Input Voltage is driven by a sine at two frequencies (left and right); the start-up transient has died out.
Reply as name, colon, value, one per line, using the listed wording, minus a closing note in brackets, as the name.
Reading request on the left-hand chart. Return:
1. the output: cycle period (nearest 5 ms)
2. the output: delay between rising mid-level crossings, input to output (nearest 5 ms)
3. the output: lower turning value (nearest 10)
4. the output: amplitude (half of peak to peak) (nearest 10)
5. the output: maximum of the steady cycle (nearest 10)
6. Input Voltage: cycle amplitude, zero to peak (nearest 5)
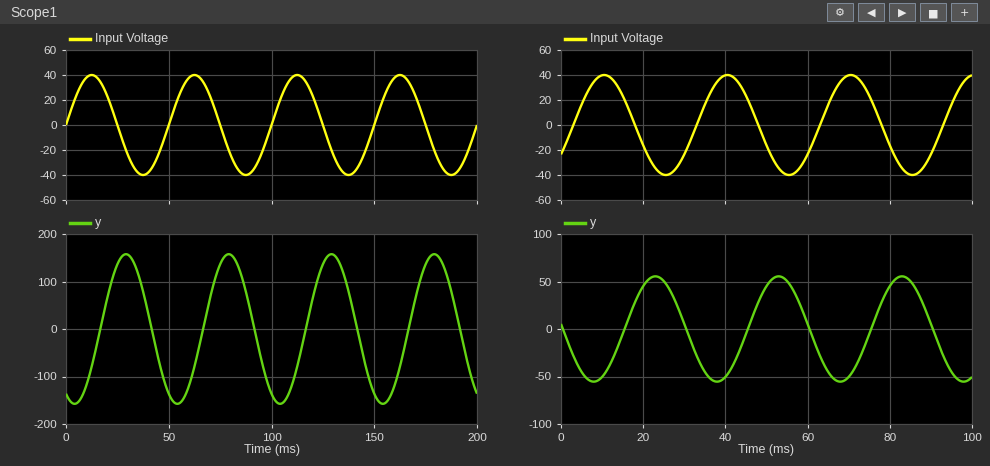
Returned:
the output: cycle period: 50 ms
the output: delay between rising mid-level crossings, input to output: 15 ms
the output: lower turning value: -160
the output: amplitude (half of peak to peak): 160
the output: maximum of the steady cycle: 160
Input Voltage: cycle amplitude, zero to peak: 40
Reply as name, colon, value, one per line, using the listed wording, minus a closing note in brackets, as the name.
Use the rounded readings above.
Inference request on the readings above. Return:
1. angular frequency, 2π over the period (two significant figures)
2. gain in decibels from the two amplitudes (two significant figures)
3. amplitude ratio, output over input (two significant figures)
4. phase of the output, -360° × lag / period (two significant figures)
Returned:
angular frequency, 2π over the period: 0.13 rad/ms
gain in decibels from the two amplitudes: 12 dB
amplitude ratio, output over input: 4.0
phase of the output, -360° × lag / period: -110°
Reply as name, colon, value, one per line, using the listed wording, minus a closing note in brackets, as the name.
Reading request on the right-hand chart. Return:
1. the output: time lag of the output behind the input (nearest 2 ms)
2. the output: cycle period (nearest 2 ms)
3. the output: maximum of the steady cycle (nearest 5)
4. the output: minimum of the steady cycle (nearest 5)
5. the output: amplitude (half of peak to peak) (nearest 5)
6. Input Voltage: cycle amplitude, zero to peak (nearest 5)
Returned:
the output: time lag of the output behind the input: 12 ms
the output: cycle period: 30 ms
the output: maximum of the steady cycle: 55
the output: minimum of the steady cycle: -55
the output: amplitude (half of peak to peak): 55
Input Voltage: cycle amplitude, zero to peak: 40
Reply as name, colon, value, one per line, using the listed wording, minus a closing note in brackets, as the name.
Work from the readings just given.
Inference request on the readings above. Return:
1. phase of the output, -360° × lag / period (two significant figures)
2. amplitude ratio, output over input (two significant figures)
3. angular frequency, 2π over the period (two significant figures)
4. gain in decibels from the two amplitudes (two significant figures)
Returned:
phase of the output, -360° × lag / period: -140°
amplitude ratio, output over input: 1.4
angular frequency, 2π over the period: 0.21 rad/ms
gain in decibels from the two amplitudes: 2.8 dB
